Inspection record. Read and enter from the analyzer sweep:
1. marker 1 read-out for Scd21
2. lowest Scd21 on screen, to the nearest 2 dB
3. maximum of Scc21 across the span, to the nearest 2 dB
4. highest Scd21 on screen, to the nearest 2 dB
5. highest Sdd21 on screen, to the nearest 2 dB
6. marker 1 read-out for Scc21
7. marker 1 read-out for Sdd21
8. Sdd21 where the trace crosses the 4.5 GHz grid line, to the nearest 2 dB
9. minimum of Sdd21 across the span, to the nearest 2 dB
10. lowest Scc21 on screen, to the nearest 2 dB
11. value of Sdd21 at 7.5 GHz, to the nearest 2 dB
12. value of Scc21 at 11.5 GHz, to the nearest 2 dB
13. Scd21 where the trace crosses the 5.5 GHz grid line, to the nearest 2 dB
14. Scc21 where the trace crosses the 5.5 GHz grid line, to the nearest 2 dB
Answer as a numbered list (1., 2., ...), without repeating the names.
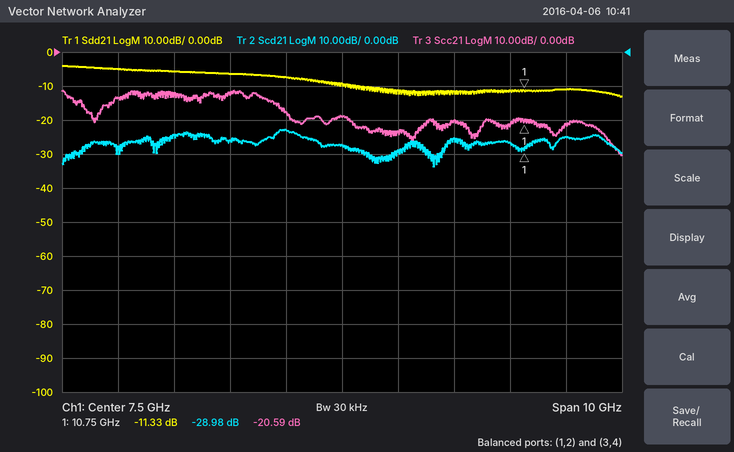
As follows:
1. -28.98 dB
2. -34 dB
3. -12 dB
4. -22 dB
5. -4 dB
6. -20.59 dB
7. -11.33 dB
8. -6 dB
9. -14 dB
10. -30 dB
11. -10 dB
12. -22 dB
13. -26 dB
14. -12 dB
